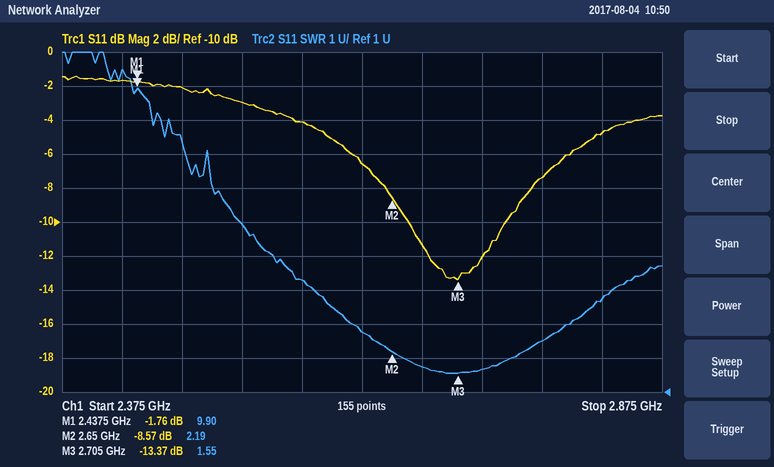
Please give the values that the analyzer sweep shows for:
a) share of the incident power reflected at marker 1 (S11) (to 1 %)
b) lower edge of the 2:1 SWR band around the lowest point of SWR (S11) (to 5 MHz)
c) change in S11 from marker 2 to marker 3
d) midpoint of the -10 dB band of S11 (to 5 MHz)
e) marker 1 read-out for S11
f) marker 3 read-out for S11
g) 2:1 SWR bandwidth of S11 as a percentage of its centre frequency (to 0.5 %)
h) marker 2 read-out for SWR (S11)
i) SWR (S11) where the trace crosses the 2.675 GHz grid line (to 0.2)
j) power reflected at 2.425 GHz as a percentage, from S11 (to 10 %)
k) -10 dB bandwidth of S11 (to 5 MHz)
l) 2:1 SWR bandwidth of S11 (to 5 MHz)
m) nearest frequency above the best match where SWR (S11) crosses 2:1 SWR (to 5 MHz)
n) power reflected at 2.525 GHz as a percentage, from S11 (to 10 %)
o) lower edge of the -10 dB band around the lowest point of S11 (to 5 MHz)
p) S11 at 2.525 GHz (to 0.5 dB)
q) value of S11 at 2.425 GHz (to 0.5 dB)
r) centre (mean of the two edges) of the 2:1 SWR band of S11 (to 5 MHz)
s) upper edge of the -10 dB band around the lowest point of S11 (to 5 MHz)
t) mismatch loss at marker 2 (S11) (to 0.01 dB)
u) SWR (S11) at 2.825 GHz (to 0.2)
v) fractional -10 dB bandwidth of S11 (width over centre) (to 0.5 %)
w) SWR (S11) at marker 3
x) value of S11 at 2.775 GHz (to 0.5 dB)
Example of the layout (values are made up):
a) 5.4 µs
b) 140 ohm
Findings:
a) 67 %
b) 2.660 GHz
c) -4.80 dB
d) 2.705 GHz
e) -1.76 dB
f) -13.37 dB
g) 3.5 %
h) 2.19
i) 1.8
j) 70 %
k) 80 MHz
l) 90 MHz
m) 2.750 GHz
n) 50 %
o) 2.665 GHz
p) -3.0 dB
q) -1.5 dB
r) 2.705 GHz
s) 2.745 GHz
t) 0.65 dB
u) 3.8
v) 3.0 %
w) 1.55
x) -7.5 dB
